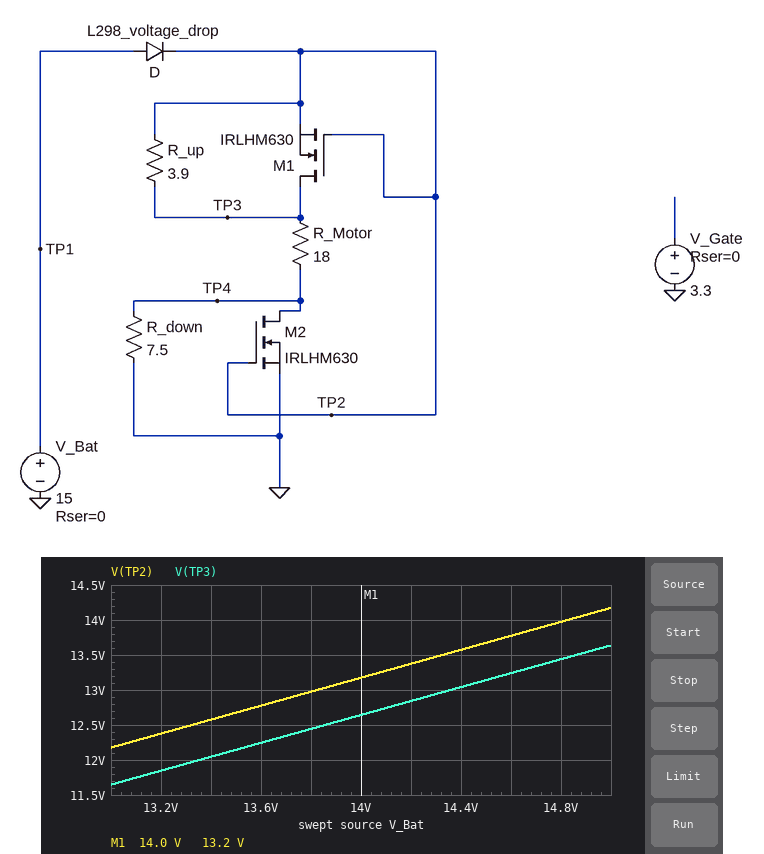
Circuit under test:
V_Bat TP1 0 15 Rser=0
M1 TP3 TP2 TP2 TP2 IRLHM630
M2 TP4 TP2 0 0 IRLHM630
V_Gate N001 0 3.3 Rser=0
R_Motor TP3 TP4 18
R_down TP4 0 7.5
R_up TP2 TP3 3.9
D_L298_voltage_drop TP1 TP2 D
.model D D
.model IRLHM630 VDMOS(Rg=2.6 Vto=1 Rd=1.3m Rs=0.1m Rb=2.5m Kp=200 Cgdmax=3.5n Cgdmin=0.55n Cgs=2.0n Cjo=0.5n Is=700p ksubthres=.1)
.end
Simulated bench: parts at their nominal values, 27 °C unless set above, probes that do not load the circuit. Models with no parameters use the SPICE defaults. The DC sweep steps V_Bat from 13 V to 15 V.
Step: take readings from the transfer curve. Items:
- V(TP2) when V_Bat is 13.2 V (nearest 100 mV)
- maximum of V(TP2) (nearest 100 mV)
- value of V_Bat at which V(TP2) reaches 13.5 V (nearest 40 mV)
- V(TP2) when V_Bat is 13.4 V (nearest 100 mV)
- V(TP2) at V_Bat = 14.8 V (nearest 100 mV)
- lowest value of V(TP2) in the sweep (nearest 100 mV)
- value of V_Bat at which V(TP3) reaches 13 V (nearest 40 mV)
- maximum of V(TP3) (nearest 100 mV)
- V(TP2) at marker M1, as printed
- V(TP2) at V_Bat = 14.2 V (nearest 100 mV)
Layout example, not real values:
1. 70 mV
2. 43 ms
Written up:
1. 12.4 V
2. 14.2 V
3. 14.32 V
4. 12.6 V
5. 14.0 V
6. 12.2 V
7. 14.36 V
8. 13.6 V
9. 13.2 V
10. 13.4 V
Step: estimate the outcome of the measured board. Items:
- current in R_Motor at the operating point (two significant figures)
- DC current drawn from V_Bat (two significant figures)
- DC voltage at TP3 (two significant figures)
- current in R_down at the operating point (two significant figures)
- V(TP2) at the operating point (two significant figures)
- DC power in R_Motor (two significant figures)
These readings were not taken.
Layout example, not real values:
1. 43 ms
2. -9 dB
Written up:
1. 760 mA
2. 760 mA
3. 14 V
4. 180 µA
5. 14 V
6. 10 W
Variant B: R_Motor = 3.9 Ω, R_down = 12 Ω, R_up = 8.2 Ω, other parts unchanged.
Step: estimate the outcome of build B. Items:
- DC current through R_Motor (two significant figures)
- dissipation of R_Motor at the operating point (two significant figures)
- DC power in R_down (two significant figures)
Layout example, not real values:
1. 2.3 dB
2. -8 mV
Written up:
1. 3.5 A
2. 47 W
3. 3.2 µW
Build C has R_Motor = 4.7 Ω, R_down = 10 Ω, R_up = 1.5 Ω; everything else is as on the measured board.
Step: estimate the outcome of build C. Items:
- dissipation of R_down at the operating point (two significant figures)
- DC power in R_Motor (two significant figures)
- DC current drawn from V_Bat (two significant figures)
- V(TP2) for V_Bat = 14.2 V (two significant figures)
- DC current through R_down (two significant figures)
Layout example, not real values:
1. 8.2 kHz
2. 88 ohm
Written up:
1. 2.6 µW
2. 39 W
3. 2.9 A
4. 13 V
5. 510 µA
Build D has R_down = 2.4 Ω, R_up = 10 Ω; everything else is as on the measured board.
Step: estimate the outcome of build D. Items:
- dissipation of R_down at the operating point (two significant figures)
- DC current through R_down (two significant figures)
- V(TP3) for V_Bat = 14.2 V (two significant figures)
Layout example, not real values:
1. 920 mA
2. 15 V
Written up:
1. 760 nW
2. 560 µA
3. 13 V
